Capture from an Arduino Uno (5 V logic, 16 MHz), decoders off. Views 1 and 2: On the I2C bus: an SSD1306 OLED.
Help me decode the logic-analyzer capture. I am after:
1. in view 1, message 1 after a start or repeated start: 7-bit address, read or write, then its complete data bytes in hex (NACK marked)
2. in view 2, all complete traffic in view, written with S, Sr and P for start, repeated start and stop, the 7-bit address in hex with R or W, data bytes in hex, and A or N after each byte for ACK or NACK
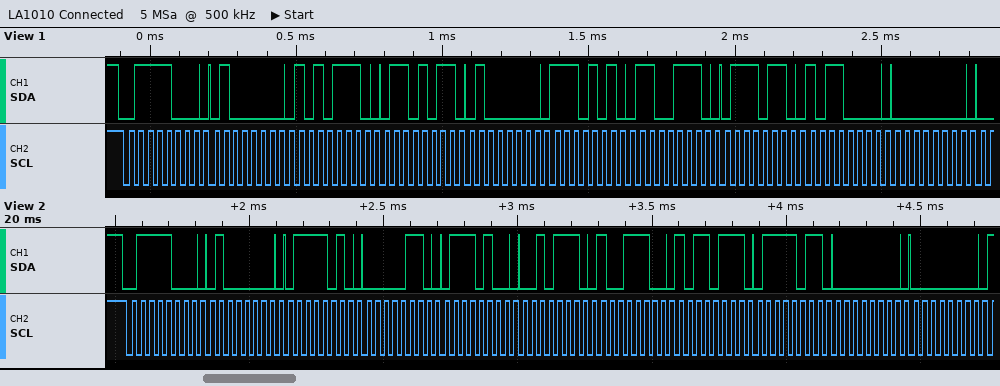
0x3C write: 40 AE 6B 40 EA CE 76 B0 00
S 3CW A 40 A 7A A 06 A 74 A 2E A 9C A B7 A 7B A 00 A 00 A
